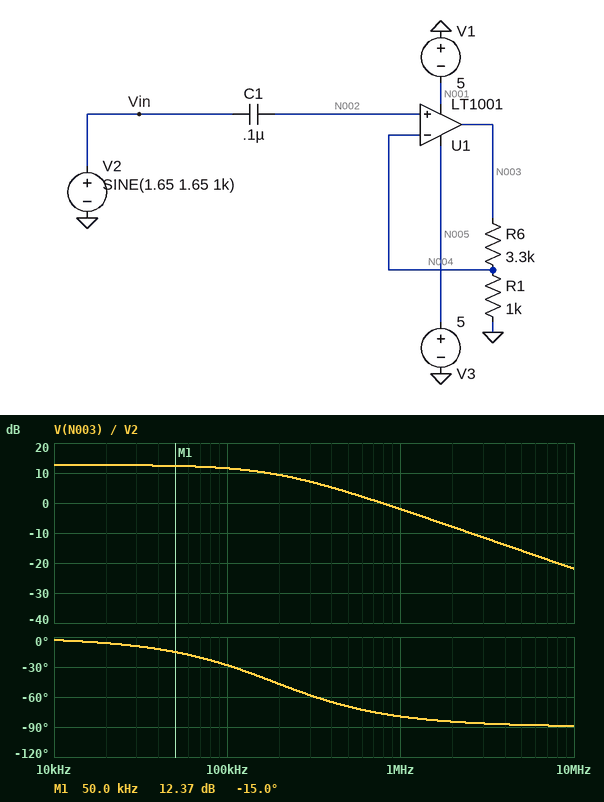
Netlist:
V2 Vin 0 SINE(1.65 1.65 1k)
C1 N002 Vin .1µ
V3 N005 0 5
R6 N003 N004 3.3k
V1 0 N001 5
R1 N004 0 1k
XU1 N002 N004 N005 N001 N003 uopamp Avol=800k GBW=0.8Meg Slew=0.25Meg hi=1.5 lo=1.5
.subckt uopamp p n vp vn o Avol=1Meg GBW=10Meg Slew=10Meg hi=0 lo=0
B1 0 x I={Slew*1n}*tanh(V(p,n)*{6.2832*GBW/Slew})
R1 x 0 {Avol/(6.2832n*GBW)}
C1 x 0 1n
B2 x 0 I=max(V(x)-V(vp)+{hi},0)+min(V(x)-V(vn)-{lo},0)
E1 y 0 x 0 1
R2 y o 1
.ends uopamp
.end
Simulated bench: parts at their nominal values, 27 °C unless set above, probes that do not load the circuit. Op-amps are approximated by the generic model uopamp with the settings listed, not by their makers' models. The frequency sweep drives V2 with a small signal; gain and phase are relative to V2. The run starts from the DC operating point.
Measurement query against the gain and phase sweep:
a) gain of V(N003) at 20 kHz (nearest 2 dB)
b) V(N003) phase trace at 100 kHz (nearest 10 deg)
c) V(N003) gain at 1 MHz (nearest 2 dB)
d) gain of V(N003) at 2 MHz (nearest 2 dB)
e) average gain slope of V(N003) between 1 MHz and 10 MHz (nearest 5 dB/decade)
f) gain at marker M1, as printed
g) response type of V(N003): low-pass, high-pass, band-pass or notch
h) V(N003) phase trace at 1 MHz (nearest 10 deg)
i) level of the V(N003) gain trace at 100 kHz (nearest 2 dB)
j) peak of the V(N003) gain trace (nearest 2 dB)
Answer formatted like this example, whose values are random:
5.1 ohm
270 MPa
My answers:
12 dB
-30 deg
-2 dB
-8 dB
-20 dB/decade
12.37 dB
low-pass
-80 deg
12 dB
12 dB
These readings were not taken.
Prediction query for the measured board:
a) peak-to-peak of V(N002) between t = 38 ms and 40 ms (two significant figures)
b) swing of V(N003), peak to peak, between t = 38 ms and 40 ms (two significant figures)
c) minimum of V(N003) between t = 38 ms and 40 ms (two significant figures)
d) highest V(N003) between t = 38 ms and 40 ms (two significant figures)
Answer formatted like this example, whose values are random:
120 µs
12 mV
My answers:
3.3 V
7.0 V
-3.5 V
3.5 V
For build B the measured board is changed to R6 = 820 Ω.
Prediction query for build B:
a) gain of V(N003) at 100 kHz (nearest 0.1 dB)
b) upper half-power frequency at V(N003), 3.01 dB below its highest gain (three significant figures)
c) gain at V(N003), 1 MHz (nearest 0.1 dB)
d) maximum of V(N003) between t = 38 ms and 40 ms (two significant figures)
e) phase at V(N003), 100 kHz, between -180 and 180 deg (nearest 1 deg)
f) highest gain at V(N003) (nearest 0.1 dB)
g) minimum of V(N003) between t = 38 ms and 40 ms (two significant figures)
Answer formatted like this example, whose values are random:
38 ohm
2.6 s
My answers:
5.0 dB
439 kHz
-2.7 dB
3.0 V
-13 deg
5.2 dB
-3.0 V
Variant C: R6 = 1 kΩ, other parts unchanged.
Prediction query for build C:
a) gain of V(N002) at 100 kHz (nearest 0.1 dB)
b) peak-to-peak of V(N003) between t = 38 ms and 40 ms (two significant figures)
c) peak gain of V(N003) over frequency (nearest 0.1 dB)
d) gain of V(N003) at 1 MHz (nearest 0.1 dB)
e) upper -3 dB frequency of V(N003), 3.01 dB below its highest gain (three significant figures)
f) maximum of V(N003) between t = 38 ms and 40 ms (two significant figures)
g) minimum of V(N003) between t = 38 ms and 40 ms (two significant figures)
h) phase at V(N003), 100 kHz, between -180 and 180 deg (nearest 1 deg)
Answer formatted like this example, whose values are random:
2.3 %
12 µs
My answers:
0 dB
6.6 V
6.0 dB
-2.6 dB
400 kHz
3.3 V
-3.3 V
-14 deg
